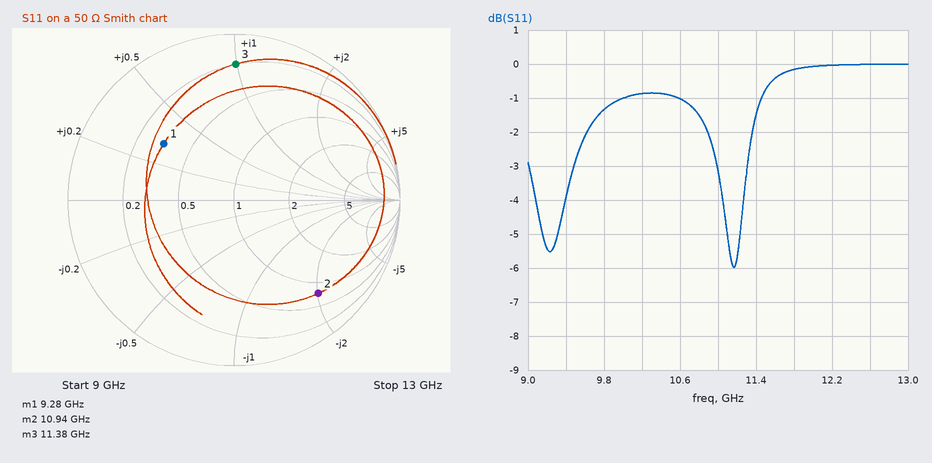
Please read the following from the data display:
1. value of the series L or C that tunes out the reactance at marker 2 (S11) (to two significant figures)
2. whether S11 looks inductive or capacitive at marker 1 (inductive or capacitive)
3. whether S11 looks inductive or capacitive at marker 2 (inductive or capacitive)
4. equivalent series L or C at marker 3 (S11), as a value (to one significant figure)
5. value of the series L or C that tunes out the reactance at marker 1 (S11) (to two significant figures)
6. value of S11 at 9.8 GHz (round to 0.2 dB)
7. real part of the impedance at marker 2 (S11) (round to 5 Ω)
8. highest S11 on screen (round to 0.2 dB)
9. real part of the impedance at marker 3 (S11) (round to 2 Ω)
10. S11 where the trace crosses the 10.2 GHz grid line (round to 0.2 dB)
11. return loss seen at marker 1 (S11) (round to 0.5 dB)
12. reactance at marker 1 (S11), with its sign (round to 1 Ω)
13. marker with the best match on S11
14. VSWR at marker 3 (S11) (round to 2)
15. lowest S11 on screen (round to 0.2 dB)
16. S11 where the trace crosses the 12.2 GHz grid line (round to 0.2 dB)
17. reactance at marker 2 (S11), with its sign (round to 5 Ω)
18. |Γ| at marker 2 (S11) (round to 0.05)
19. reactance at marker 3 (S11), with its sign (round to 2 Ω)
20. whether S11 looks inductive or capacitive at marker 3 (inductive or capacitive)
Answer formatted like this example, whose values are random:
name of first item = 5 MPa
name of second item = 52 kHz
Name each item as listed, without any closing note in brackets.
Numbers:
value of the series L or C that tunes out the reactance at marker 2 (S11) = 1.5 nH
whether S11 looks inductive or capacitive at marker 1 = inductive
whether S11 looks inductive or capacitive at marker 2 = capacitive
equivalent series L or C at marker 3 (S11), as a value = 700 pH
value of the series L or C that tunes out the reactance at marker 1 (S11) = 1.1 pF
value of S11 at 9.8 GHz = -1.4 dB
real part of the impedance at marker 2 (S11) = 40 Ω
highest S11 on screen = 0.0 dB
real part of the impedance at marker 3 (S11) = 10 Ω
S11 where the trace crosses the 10.2 GHz grid line = -0.8 dB
return loss seen at marker 1 (S11) = 5.5 dB
reactance at marker 1 (S11), with its sign = +16 Ω
marker with the best match on S11 = marker 1
VSWR at marker 3 (S11) = 10
lowest S11 on screen = -6.0 dB
S11 where the trace crosses the 12.2 GHz grid line = 0.0 dB
reactance at marker 2 (S11), with its sign = -100 Ω
|Γ| at marker 2 (S11) = 0.75
reactance at marker 3 (S11), with its sign = +50 Ω
whether S11 looks inductive or capacitive at marker 3 = inductive
